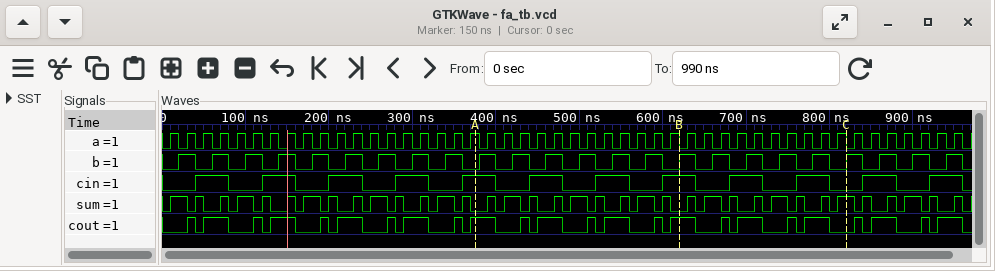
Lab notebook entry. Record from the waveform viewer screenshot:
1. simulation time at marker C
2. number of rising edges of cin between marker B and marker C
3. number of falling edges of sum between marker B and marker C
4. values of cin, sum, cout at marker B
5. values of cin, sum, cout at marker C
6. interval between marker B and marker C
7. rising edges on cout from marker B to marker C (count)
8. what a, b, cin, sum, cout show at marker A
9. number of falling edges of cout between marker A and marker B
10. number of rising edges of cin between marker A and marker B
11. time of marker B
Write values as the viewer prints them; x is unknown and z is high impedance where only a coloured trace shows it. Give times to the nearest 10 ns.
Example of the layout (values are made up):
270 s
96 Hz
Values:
820 ns
2
7
cin=1, sum=0, cout=1
cin=0, sum=1, cout=0
200 ns
4
a=1, b=0, cin=1, sum=0, cout=1
6
3
620 ns
